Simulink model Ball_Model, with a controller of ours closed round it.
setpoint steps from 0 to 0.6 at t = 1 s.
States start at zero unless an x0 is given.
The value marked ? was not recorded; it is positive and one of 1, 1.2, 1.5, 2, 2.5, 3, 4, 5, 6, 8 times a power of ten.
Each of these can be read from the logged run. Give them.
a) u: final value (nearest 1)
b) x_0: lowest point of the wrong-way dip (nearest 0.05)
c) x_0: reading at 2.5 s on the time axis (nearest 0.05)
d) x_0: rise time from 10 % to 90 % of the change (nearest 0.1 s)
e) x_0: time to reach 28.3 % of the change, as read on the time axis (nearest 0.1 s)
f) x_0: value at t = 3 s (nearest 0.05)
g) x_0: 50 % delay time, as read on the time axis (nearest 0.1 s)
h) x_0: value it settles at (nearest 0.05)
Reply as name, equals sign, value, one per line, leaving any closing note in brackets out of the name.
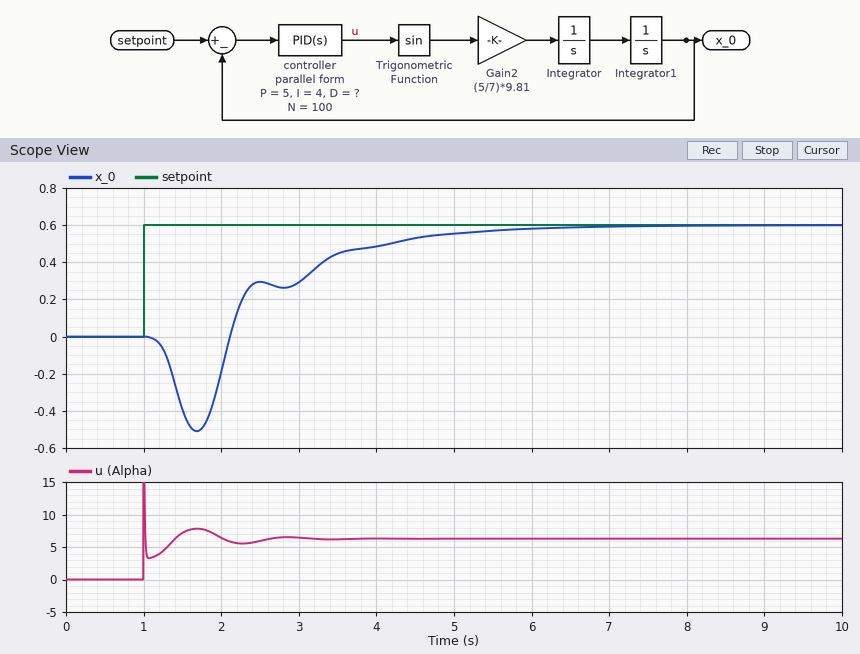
u: final value = 6
x_0: lowest point of the wrong-way dip = -0.50
x_0: reading at 2.5 s on the time axis = 0.30
x_0: rise time from 10 % to 90 % of the change = 2.5 s
x_0: time to reach 28.3 % of the change, as read on the time axis = 2.2 s
x_0: value at t = 3 s = 0.30
x_0: 50 % delay time, as read on the time axis = 3.0 s
x_0: value it settles at = 0.60
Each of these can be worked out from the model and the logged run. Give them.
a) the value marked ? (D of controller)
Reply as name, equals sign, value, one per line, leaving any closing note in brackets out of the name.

the value marked ? = 0.6
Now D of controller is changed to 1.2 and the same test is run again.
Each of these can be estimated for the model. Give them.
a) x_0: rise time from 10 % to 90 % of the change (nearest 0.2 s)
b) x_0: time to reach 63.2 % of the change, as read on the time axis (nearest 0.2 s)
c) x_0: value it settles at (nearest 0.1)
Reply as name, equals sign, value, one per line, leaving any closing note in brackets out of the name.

x_0: rise time from 10 % to 90 % of the change = 2.2 s
x_0: time to reach 63.2 % of the change, as read on the time axis = 3.2 s
x_0: value it settles at = 0.6
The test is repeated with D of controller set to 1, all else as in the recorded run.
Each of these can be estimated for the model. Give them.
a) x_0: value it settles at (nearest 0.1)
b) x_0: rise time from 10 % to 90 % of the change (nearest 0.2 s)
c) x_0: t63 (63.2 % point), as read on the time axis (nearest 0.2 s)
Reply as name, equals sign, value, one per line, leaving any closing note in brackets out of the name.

x_0: value it settles at = 0.6
x_0: rise time from 10 % to 90 % of the change = 2.2 s
x_0: t63 (63.2 % point), as read on the time axis = 3.2 s
